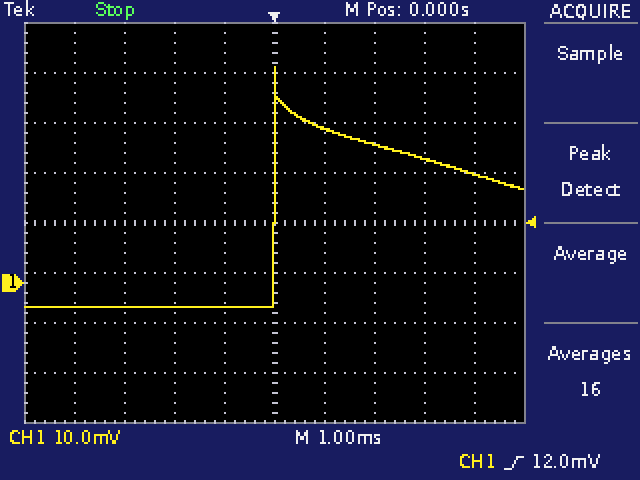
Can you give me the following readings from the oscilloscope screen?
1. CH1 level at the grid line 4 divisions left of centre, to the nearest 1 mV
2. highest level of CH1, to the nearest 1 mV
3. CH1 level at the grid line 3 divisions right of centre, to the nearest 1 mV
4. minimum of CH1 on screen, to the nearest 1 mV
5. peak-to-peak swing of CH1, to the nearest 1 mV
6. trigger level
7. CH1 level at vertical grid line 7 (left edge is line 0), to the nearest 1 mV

-5 mV
43 mV
25 mV
-5 mV
48 mV
12.0 mV
28 mV
